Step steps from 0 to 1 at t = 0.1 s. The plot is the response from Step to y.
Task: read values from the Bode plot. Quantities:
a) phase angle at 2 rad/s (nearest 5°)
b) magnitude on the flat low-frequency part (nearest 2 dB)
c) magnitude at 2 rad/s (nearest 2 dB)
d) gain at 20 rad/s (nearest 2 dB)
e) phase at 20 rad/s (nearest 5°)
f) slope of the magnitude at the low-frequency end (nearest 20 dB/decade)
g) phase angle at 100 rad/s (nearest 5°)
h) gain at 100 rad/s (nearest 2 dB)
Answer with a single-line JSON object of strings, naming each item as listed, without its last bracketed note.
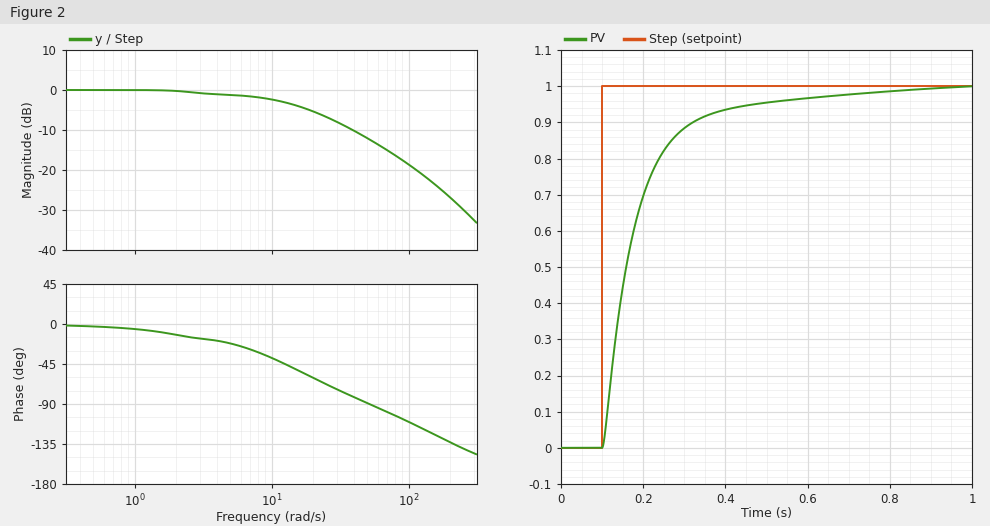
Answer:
{"phase angle at 2 rad/s": "-10°", "magnitude on the flat low-frequency part": "0 dB", "magnitude at 2 rad/s": "0 dB", "gain at 20 rad/s": "-6 dB", "phase at 20 rad/s": "-60°", "slope of the magnitude at the low-frequency end": "0 dB/decade", "phase angle at 100 rad/s": "-110°", "gain at 100 rad/s": "-18 dB"}
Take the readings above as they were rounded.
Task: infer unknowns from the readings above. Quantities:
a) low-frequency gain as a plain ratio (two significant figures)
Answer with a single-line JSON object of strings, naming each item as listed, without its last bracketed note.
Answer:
{"low-frequency gain as a plain ratio": "1.0"}
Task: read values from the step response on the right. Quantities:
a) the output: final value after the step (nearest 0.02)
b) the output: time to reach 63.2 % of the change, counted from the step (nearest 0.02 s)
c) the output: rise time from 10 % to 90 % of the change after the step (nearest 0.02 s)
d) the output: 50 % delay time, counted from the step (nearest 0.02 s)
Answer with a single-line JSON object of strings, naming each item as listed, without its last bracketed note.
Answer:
{"the output: final value after the step": "1.00", "the output: time to reach 63.2 % of the change, counted from the step": "0.08 s", "the output: rise time from 10 % to 90 % of the change after the step": "0.20 s", "the output: 50 % delay time, counted from the step": "0.06 s"}
